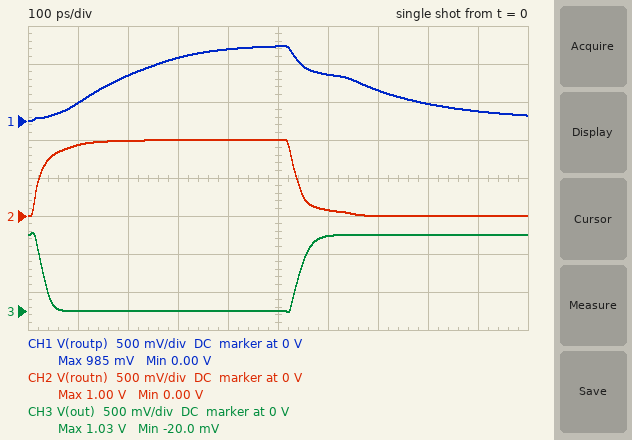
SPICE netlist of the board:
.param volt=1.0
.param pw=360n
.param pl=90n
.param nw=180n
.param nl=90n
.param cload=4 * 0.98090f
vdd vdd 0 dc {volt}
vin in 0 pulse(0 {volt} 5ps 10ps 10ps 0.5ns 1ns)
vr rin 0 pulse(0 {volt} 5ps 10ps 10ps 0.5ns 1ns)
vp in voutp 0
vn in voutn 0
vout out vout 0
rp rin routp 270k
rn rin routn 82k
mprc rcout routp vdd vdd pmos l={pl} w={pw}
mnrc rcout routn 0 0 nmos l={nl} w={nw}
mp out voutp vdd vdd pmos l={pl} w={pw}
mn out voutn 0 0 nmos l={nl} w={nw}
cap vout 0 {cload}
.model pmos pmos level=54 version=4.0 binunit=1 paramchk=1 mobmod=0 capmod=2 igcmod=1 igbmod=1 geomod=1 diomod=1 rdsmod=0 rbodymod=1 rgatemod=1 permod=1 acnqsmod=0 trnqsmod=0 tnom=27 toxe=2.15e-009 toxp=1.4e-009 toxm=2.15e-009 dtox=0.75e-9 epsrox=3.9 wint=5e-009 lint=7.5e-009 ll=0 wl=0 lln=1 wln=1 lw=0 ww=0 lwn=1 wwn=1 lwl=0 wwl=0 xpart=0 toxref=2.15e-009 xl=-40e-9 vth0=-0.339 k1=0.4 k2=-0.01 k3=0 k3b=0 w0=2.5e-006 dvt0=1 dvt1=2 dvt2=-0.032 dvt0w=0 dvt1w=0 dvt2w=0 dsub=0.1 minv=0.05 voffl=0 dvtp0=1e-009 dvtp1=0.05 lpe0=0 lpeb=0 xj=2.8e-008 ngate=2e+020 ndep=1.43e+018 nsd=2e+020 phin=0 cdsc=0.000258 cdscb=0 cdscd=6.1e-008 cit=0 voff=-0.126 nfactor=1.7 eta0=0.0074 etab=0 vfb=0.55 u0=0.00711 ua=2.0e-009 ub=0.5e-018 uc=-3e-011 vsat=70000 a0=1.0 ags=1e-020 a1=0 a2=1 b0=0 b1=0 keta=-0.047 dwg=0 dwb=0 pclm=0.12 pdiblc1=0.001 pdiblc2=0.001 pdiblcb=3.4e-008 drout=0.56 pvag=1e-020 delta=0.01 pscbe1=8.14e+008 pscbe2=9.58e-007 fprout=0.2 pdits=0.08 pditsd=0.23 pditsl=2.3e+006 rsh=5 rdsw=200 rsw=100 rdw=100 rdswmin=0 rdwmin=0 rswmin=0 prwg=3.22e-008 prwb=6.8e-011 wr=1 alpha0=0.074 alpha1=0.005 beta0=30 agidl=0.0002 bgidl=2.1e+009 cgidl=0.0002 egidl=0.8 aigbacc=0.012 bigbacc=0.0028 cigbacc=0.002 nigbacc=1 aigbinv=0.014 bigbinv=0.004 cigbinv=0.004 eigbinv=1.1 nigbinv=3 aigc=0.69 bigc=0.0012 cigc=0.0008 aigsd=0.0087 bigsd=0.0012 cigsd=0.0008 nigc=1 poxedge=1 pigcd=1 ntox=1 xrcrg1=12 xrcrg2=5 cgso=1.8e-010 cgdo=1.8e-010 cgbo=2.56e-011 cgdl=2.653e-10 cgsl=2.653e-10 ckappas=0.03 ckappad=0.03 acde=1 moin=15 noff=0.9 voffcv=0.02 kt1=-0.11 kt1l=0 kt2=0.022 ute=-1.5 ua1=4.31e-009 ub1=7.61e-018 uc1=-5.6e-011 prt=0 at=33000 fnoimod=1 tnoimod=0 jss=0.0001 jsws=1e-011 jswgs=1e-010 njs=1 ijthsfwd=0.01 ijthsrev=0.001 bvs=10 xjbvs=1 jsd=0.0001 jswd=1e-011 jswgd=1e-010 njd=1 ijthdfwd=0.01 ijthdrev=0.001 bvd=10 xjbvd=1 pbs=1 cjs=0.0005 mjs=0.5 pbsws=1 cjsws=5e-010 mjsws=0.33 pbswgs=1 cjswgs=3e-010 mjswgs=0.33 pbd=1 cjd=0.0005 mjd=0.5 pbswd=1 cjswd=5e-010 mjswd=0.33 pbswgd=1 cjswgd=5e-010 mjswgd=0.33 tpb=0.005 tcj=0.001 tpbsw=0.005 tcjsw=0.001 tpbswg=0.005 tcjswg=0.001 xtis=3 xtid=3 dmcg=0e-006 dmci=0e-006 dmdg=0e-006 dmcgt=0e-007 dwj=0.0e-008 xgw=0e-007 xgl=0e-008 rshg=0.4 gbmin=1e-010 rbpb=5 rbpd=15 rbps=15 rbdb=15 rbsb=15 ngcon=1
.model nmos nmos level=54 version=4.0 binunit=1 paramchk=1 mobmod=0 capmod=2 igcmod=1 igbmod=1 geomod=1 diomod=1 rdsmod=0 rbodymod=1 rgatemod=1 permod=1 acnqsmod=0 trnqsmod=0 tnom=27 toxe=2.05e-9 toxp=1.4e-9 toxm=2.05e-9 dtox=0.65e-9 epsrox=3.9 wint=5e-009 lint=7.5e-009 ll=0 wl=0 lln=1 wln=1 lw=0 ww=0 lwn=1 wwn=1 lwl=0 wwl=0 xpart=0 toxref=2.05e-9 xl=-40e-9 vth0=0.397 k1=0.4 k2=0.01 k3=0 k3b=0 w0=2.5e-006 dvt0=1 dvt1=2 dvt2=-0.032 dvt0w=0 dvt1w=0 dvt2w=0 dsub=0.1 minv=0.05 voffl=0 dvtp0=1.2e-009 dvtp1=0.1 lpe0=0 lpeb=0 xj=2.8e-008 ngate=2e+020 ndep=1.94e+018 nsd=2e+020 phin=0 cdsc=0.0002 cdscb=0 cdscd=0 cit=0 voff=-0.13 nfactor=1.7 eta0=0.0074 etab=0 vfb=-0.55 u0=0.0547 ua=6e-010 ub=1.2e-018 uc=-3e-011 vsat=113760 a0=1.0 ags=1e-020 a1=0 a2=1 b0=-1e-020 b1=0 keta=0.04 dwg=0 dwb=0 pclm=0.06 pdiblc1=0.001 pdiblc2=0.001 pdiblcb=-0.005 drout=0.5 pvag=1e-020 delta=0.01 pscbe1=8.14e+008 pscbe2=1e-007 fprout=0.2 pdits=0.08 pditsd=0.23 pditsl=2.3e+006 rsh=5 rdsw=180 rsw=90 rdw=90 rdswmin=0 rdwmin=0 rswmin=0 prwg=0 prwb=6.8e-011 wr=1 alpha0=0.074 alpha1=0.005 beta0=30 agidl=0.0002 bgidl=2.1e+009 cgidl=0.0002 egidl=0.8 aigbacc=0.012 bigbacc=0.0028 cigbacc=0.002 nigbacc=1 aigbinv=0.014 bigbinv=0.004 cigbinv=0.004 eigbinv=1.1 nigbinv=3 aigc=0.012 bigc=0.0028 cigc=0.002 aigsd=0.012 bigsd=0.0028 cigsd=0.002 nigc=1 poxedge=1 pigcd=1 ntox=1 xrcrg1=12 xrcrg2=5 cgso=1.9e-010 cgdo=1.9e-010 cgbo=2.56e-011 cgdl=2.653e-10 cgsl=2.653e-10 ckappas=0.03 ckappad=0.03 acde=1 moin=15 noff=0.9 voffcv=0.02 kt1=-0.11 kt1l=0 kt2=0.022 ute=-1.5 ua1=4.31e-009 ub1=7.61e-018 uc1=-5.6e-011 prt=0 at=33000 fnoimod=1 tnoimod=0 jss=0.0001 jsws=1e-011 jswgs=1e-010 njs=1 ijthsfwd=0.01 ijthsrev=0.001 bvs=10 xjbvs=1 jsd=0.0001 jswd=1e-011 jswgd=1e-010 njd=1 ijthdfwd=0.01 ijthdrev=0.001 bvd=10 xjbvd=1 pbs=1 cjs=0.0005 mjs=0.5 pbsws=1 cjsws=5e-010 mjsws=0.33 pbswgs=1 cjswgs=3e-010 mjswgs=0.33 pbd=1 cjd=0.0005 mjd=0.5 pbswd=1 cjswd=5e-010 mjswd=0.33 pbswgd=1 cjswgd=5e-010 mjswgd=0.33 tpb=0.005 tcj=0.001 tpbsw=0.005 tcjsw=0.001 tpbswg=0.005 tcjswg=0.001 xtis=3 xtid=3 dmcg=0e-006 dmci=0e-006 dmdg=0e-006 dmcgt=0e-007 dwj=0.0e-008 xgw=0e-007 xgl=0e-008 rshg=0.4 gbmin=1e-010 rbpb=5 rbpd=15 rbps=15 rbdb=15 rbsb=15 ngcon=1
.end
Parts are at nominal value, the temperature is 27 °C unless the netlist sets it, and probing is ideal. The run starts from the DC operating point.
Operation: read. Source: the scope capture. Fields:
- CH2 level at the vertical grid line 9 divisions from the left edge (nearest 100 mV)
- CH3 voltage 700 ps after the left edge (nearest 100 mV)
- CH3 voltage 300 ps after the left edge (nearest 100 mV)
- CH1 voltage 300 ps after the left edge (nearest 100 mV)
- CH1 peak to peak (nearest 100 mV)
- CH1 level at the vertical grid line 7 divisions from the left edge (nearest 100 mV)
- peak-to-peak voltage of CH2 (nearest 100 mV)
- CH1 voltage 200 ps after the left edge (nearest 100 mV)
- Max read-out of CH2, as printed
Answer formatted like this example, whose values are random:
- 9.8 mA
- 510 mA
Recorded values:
- 0 V
- 1.0 V
- 0 V
- 800 mV
- 1.0 V
- 400 mV
- 1.0 V
- 600 mV
- 1.00 V
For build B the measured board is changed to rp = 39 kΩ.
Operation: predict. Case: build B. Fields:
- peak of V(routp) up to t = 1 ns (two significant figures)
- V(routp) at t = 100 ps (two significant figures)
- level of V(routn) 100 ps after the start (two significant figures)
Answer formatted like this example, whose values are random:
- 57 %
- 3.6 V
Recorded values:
- 1.0 V
- 990 mV
- 960 mV
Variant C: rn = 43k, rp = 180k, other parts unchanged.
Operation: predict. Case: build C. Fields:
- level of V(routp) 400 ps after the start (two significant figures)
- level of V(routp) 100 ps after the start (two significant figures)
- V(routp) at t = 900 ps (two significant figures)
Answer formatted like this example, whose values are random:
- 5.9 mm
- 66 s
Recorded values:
- 990 mV
- 420 mV
- 44 mV
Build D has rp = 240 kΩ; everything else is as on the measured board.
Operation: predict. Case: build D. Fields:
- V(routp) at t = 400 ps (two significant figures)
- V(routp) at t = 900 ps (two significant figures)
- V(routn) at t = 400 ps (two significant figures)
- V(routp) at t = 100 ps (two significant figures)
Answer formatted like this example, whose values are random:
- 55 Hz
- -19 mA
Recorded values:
- 970 mV
- 97 mV
- 1.0 V
- 280 mV
